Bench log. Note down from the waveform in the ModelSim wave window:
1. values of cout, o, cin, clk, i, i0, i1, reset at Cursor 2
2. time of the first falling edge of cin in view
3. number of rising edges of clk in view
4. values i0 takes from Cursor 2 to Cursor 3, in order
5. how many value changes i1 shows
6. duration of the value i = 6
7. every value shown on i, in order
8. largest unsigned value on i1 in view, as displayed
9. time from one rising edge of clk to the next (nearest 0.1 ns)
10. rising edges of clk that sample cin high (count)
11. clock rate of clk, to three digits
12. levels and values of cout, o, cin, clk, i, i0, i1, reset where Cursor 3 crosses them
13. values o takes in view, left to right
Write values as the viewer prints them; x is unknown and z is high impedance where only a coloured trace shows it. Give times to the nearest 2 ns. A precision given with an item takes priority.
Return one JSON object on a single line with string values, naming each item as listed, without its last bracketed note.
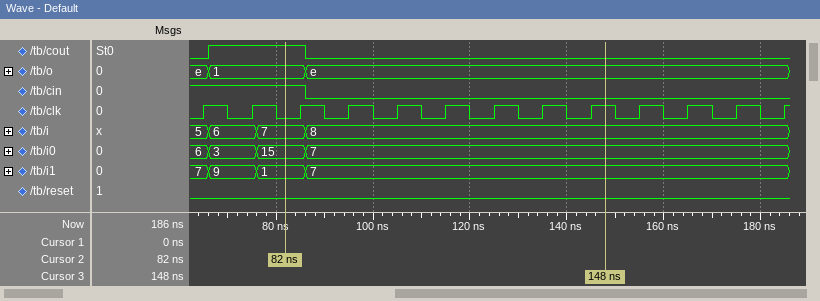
{"values of cout, o, cin, clk, i, i0, i1, reset at Cursor 2": "cout=1, o=1, cin=1, clk=0, i=7, i0=15, i1=1, reset=0", "time of the first falling edge of cin in view": "86 ns", "number of rising edges of clk in view": "13", "values i0 takes from Cursor 2 to Cursor 3, in order": "15, 7", "how many value changes i1 shows": "3", "duration of the value i = 6": "10 ns", "every value shown on i, in order": "5, 6, 7, 8", "largest unsigned value on i1 in view, as displayed": "9", "time from one rising edge of clk to the next": "10 ns", "rising edges of clk that sample cin high": "3", "clock rate of clk, to three digits": "100 MHz", "levels and values of cout, o, cin, clk, i, i0, i1, reset where Cursor 3 crosses them": "cout=0, o=e, cin=0, clk=1, i=8, i0=7, i1=7, reset=0", "values o takes in view, left to right": "e, 1, e"}
